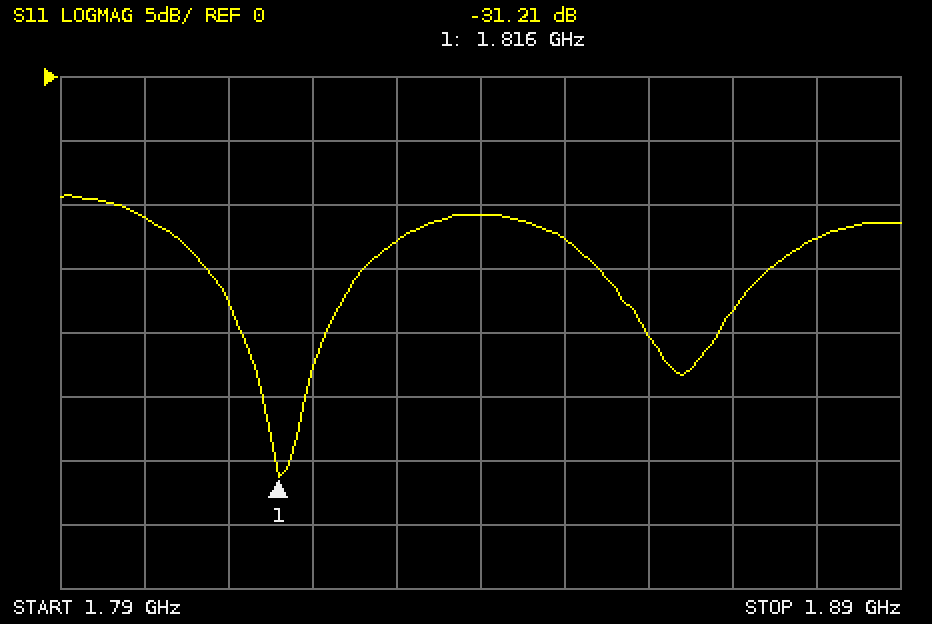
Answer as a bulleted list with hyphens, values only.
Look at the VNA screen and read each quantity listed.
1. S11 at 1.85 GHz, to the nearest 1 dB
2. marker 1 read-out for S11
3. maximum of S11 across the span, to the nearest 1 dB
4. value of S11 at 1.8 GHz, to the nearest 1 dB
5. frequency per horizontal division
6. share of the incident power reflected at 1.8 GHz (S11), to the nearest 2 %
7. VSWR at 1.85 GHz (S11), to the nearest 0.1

- -13 dB
- -31.21 dB
- -9 dB
- -11 dB
- 10 MHz
- 8 %
- 1.6
